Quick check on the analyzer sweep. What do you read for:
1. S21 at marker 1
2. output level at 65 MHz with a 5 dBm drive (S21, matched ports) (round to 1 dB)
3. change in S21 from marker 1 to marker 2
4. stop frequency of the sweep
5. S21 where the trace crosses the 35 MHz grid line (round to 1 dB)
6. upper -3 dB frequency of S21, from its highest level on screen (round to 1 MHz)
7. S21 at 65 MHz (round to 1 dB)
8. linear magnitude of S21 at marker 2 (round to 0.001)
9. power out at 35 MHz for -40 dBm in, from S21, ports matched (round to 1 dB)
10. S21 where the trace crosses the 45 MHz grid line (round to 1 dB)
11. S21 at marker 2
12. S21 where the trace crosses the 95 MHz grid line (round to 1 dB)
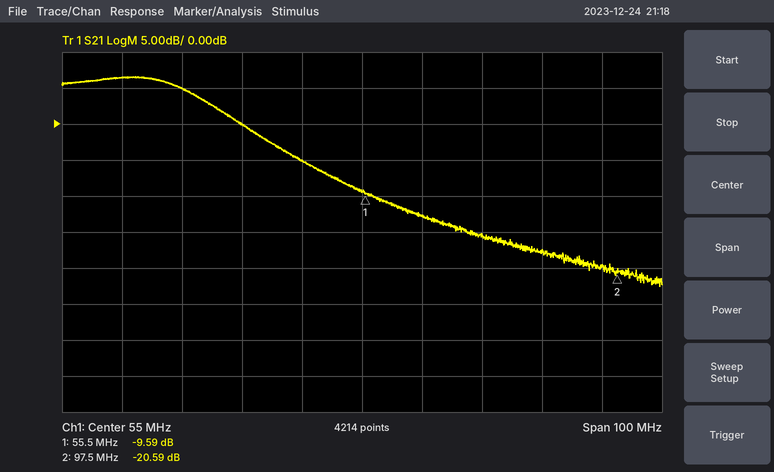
-9.59 dB
-8 dBm
-11.00 dB
105 MHz
0 dB
28 MHz
-13 dB
0.093
-40 dBm
-5 dB
-20.59 dB
-20 dB
